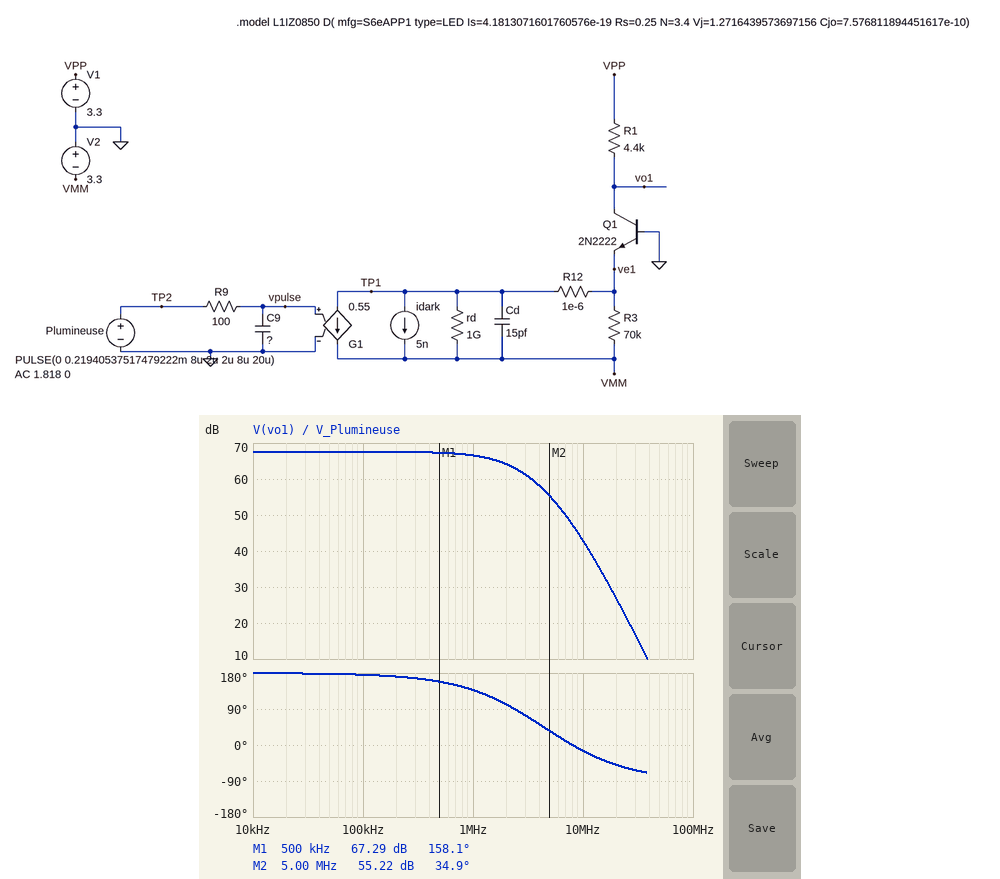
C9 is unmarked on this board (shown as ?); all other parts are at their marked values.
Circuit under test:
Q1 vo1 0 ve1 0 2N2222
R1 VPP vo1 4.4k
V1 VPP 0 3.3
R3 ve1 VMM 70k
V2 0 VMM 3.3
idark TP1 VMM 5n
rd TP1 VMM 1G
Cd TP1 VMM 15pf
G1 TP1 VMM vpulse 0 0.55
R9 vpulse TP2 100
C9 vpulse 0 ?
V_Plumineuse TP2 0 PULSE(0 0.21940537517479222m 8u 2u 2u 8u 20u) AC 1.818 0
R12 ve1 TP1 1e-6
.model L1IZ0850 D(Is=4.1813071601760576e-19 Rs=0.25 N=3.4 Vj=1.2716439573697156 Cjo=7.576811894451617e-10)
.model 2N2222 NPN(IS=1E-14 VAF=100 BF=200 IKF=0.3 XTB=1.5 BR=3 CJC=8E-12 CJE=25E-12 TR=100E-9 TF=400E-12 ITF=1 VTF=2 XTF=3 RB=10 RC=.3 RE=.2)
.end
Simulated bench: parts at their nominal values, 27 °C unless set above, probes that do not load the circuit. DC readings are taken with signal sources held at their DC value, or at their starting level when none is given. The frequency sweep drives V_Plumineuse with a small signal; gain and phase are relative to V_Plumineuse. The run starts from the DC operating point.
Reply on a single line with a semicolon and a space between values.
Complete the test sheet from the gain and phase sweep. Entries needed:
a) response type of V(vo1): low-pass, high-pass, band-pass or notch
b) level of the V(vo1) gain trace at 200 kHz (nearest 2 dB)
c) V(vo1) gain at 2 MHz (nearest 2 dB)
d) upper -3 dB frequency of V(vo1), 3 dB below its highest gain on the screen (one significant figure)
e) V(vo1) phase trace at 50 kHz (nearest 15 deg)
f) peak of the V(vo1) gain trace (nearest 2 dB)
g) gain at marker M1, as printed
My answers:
low-pass; 68 dB; 64 dB; 2 MHz; 180 deg; 68 dB; 67.29 dB
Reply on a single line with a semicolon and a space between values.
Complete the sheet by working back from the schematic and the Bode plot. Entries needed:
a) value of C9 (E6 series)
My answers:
680 pF
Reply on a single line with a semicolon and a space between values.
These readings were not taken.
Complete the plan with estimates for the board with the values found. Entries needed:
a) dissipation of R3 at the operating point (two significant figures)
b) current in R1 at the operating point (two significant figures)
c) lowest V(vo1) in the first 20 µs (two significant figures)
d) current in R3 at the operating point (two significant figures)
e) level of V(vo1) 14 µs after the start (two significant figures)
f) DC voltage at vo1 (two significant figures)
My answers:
110 µW; 39 µA; 2.6 V; 39 µA; 2.6 V; 3.1 V
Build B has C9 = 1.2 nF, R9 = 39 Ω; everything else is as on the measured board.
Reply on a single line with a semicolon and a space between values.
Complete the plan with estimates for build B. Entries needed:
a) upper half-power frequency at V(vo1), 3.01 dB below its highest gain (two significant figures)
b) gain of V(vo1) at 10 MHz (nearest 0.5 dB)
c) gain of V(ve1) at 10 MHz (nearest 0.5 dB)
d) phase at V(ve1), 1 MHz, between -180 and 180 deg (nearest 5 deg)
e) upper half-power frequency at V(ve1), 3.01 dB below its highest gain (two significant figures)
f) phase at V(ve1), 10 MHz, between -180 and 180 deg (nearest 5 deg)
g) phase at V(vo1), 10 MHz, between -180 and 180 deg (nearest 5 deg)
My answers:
2.3 MHz; 46.0 dB; 34.0 dB; 150 deg; 2.5 MHz; 45 deg; -10 deg
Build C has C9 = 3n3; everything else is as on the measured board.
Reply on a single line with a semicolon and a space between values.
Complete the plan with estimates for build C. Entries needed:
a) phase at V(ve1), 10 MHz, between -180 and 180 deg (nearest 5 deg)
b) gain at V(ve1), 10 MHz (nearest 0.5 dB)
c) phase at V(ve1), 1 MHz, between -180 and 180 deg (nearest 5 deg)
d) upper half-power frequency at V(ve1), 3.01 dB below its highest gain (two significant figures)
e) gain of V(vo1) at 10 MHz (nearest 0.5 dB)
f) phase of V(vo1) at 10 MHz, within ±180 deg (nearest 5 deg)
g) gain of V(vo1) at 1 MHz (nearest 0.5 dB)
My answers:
30 deg; 17.5 dB; 105 deg; 480 kHz; 29.5 dB; -25 deg; 60.0 dB
